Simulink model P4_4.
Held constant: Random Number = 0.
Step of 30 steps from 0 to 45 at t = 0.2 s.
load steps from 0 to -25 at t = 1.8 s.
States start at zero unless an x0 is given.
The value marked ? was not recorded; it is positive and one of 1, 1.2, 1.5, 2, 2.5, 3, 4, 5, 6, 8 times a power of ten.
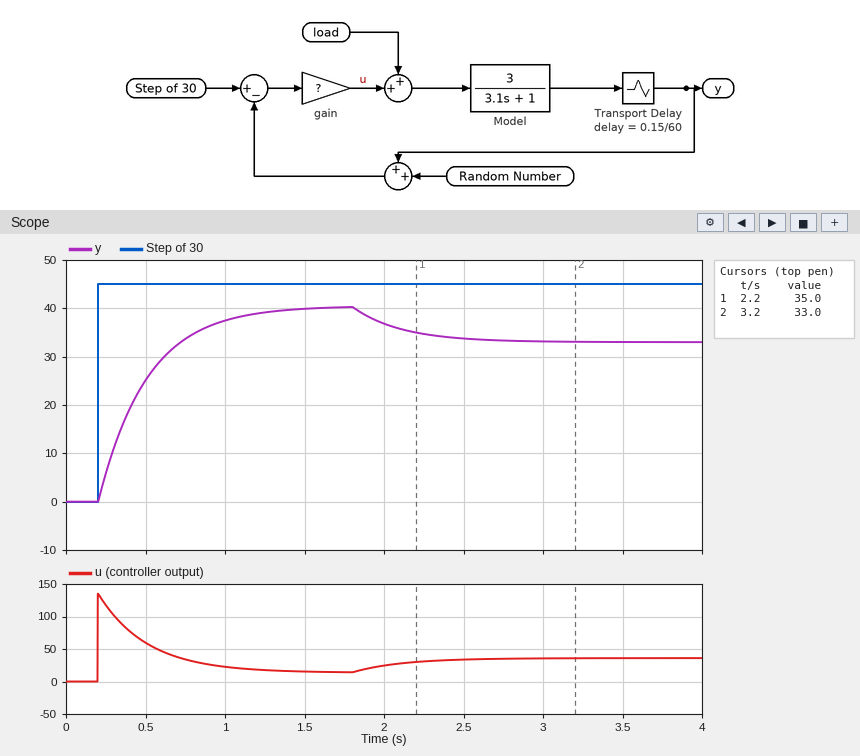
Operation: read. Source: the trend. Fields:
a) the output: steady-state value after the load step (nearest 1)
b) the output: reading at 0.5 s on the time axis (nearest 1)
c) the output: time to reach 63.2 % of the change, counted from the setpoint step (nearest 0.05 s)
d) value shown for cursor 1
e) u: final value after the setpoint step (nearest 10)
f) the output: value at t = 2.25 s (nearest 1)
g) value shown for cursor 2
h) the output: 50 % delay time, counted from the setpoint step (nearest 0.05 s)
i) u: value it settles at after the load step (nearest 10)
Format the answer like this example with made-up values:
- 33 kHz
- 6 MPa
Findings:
- 33
- 25
- 0.30 s
- 35.0
- 10
- 35
- 33.0
- 0.20 s
- 40
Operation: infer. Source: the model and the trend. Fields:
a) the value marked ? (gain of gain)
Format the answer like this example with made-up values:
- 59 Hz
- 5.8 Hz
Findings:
- 3
